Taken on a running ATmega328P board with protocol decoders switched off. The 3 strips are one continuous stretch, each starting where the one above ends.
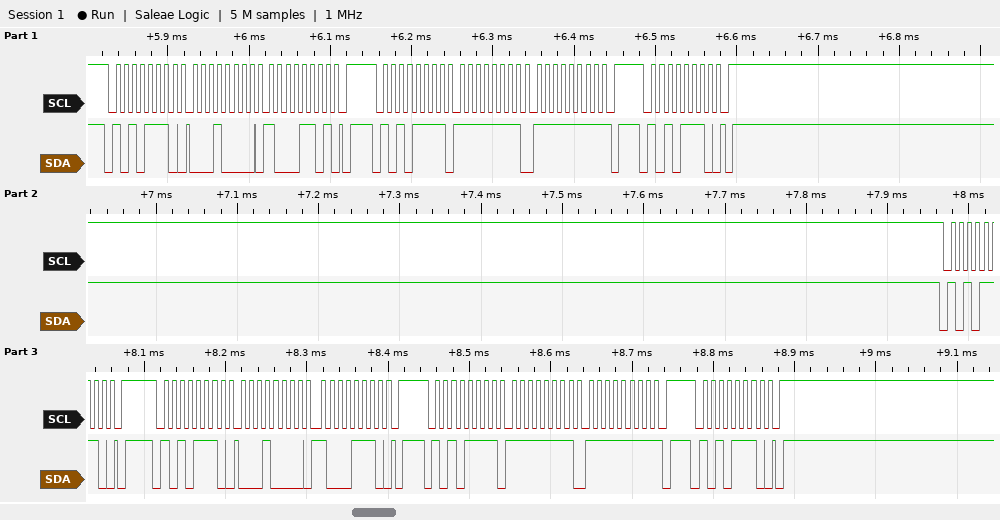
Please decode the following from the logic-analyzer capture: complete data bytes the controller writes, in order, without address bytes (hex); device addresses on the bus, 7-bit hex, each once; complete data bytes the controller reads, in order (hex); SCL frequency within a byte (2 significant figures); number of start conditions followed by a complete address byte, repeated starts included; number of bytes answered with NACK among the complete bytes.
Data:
10 8D 10 8E
0x57
FF FF FF FF
100 kHz
7
2
